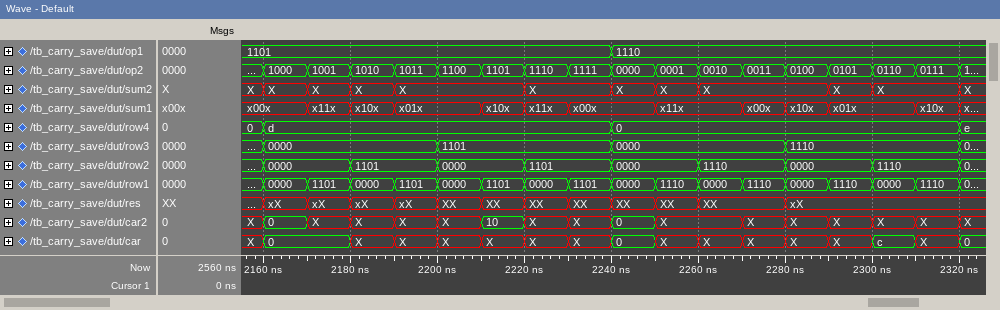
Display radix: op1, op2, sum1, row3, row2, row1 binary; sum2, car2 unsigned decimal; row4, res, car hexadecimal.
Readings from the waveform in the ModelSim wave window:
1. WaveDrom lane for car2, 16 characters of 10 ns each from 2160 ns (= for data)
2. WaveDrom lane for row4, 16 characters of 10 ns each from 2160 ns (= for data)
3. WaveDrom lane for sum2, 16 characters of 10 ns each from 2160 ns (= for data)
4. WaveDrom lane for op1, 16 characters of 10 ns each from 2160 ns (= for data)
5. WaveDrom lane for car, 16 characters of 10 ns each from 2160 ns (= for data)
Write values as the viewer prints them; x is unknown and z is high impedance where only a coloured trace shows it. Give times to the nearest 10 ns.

{name: 'car2', wave: '==========.=====', data: '0 X X X X 10 X X 0 X X X X X X'}
{name: 'row4', wave: '=.......=.......', data: 'd 0'}
{name: 'sum2', wave: '====..=.===..==.', data: 'X X X X X X X X X X'}
{name: 'op1', wave: '=.......=.......', data: '1101 1110'}
{name: 'car', wave: '=.==============', data: '0 X X X X X X 0 X X X X X c X'}
